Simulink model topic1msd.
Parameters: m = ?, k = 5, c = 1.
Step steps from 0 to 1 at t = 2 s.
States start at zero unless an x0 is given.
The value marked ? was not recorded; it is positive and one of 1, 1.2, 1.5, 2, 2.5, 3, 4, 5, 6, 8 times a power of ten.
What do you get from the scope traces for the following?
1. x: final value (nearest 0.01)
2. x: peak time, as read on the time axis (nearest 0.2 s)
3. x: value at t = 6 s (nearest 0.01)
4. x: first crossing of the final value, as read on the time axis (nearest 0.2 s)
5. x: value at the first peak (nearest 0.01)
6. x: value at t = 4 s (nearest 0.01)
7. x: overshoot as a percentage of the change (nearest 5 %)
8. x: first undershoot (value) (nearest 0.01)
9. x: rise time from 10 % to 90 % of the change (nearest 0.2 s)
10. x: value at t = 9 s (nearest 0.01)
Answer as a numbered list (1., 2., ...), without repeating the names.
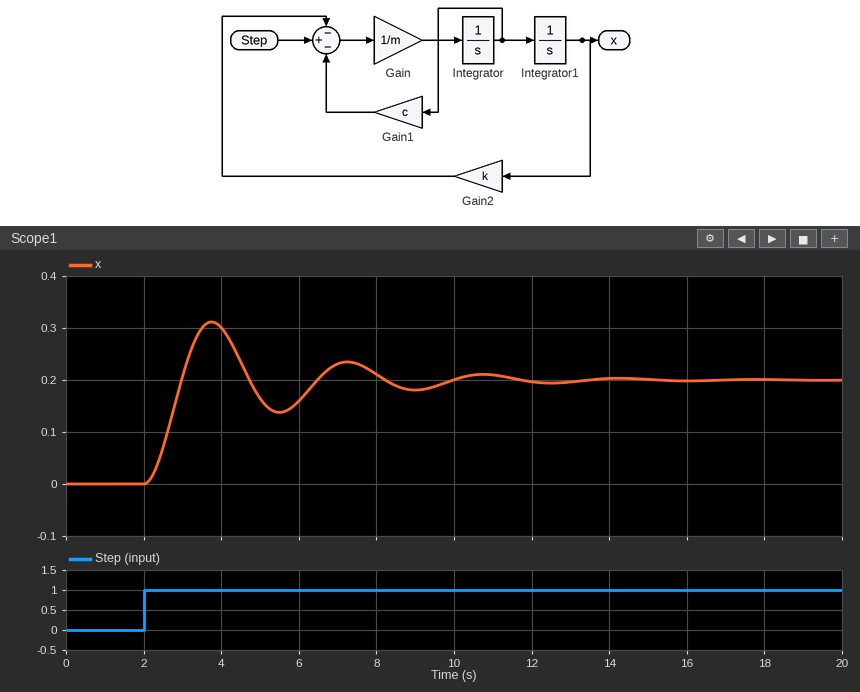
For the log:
1. 0.20
2. 3.8 s
3. 0.16
4. 3.0 s
5. 0.31
6. 0.30
7. 55 %
8. 0.14
9. 0.6 s
10. 0.18
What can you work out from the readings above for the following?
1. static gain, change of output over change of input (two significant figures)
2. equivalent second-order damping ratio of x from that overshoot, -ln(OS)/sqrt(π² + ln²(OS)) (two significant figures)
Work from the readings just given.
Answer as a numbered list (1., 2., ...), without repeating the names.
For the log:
1. 0.20
2. 0.19
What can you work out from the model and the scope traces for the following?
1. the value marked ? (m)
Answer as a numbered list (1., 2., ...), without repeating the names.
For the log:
1. 1.5
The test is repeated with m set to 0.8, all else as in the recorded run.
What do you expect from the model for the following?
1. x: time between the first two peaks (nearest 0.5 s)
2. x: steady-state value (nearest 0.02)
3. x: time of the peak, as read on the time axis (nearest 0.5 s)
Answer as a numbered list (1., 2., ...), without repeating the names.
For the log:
1. 2.5 s
2. 0.20
3. 3.5 s
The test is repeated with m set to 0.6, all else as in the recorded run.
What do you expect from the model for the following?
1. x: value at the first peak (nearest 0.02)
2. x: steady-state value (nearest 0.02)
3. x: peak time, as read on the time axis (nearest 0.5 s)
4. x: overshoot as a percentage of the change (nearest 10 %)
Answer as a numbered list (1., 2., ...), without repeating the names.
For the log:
1. 0.28
2. 0.20
3. 3.0 s
4. 40 %
